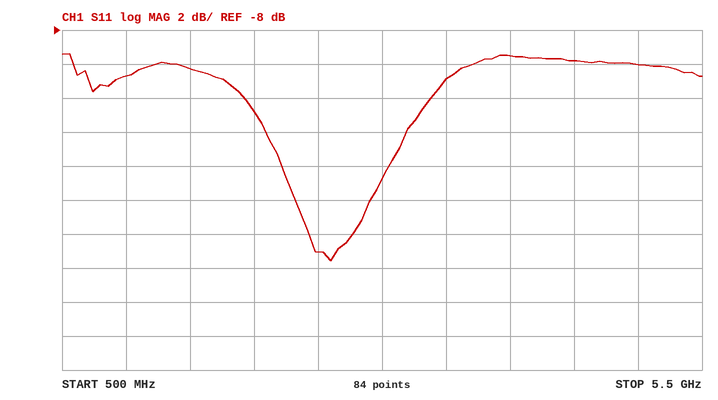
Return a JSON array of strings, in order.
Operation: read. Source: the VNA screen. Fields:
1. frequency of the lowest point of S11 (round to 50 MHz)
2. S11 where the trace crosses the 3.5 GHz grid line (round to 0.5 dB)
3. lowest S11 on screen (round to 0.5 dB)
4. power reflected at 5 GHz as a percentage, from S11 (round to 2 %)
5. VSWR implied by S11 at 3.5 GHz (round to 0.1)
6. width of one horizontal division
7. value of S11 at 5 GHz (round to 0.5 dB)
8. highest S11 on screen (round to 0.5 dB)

["2.60 GHz", "-11.0 dB", "-21.5 dB", "10 %", "1.8", "500 MHz", "-10.0 dB", "-9.5 dB"]
